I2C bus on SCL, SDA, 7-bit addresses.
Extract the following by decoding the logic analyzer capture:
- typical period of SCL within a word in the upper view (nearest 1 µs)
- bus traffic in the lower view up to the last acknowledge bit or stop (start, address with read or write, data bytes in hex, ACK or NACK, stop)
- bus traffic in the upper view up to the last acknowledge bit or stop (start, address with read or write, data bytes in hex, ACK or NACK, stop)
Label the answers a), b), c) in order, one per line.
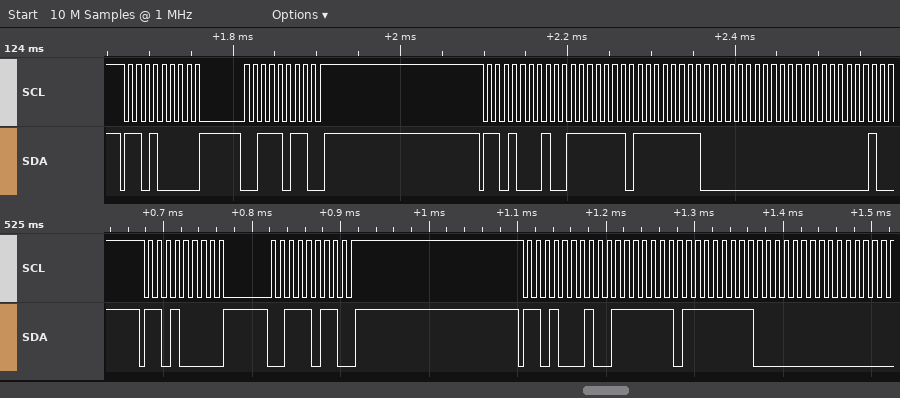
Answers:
a) 10 µs
b) start, address 68 write ACK, 3B ACK, stop, start, address 68 read ACK, 7F ACK, FF ACK, 00 ACK
c) start, address 68 write ACK, 3B ACK, stop, start, address 68 read ACK, 7F ACK, FF ACK, 00 ACK, 00 ACK
